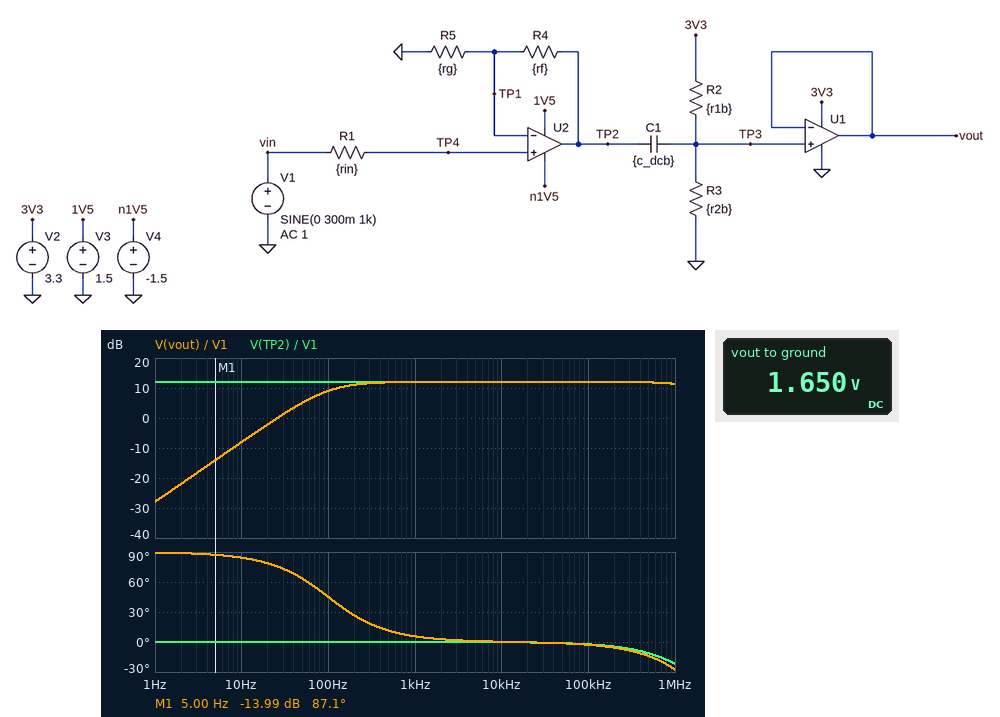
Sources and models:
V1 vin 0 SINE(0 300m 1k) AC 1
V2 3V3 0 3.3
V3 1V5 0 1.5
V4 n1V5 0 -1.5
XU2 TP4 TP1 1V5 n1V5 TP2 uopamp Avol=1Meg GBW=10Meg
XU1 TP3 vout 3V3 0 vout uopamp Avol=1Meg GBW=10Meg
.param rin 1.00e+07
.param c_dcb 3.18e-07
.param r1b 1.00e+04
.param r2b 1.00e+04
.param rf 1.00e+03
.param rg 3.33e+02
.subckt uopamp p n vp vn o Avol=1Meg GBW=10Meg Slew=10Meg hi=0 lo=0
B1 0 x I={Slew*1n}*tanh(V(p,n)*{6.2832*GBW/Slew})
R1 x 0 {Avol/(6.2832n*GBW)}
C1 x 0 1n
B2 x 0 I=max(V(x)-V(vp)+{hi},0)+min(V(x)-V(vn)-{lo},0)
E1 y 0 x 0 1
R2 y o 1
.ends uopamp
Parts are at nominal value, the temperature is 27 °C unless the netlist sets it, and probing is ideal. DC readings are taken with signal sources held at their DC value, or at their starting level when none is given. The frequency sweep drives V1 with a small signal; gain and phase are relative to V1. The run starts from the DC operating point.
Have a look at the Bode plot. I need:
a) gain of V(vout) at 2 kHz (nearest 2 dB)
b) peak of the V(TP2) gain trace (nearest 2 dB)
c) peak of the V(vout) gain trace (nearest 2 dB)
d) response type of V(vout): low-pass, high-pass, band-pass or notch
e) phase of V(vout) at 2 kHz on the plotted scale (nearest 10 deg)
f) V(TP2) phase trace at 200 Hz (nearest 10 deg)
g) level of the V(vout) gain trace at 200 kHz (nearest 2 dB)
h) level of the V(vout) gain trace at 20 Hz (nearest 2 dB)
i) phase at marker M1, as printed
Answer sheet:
12 dB
12 dB
12 dB
high-pass
0 deg
0 deg
12 dB
-2 dB
87.1 deg
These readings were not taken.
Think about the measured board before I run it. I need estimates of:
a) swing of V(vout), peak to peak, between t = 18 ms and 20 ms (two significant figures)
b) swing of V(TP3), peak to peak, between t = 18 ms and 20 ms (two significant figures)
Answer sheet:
2.4 V
2.4 V
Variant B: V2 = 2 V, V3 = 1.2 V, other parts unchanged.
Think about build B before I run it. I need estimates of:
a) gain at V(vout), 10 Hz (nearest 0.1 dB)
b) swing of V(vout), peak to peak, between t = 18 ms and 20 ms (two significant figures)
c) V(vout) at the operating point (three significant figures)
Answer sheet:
-8.0 dB
2.0 V
1.00 V
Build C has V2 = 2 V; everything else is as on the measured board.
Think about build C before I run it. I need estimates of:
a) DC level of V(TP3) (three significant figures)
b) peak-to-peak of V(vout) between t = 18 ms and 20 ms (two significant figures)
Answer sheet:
1.00 V
2.0 V
